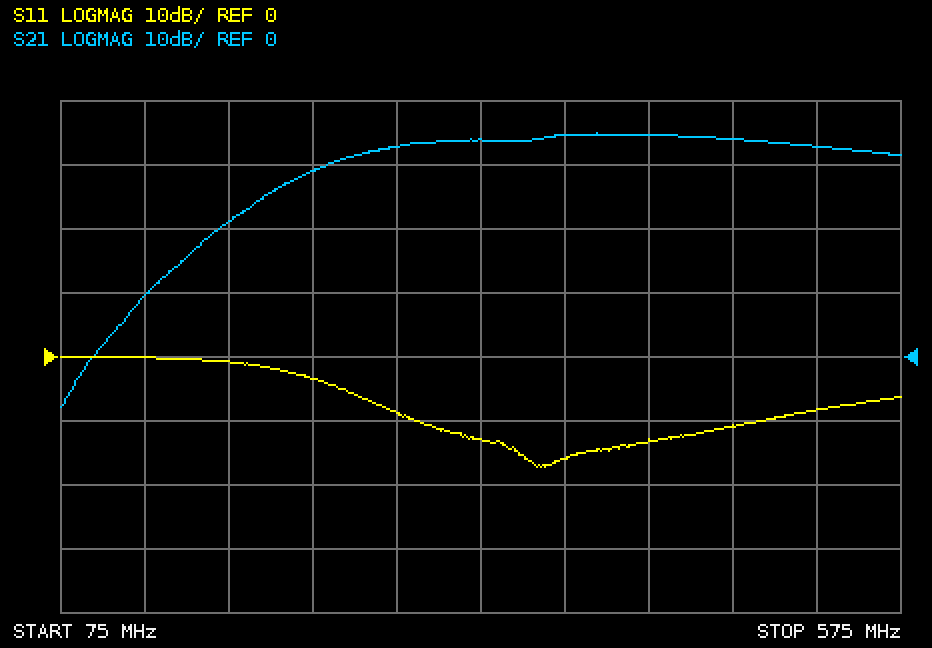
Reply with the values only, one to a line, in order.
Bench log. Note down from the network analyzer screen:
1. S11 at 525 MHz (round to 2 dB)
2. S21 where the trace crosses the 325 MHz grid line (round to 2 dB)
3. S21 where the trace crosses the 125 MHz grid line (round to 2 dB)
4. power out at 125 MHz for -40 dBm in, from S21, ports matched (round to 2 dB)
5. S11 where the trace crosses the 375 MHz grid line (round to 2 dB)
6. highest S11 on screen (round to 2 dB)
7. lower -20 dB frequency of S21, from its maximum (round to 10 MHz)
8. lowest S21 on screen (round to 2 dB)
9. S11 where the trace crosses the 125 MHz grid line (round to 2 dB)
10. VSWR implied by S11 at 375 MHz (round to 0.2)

-8 dB
34 dB
10 dB
-30 dBm
-16 dB
0 dB
150 MHz
-8 dB
0 dB
1.4
